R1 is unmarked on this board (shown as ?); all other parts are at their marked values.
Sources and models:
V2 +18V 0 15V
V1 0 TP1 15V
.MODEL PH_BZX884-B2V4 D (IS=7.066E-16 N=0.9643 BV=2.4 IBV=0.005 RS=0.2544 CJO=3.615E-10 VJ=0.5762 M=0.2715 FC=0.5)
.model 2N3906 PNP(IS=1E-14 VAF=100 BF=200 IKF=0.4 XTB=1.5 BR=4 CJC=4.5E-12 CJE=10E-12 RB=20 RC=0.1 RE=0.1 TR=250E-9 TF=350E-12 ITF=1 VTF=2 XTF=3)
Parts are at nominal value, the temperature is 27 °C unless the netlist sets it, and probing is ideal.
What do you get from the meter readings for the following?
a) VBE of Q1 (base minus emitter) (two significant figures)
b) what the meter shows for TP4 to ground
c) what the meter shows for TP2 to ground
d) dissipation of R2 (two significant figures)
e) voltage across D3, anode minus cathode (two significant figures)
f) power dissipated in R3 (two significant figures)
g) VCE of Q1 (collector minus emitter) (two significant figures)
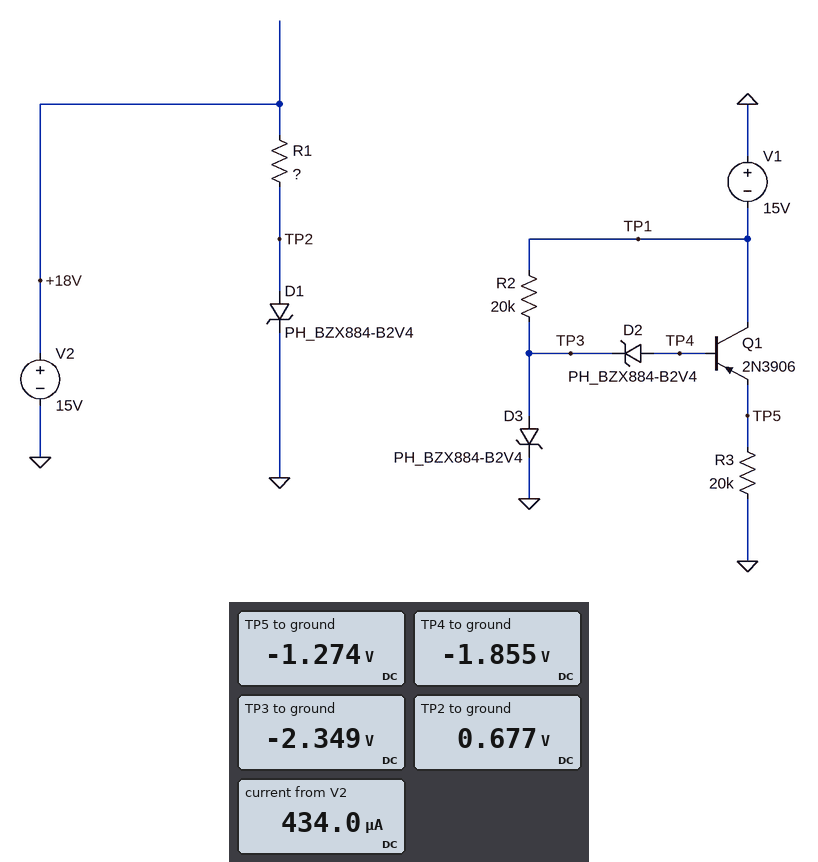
-580 mV
-1.855 V
0.677 V
8.0 mW
-2.3 V
81 µW
-14 V
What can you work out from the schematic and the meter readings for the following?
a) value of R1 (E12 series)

33 kΩ
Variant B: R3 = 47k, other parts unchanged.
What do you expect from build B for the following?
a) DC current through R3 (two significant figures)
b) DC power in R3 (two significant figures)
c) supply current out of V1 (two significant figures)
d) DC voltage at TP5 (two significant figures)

28 µA
37 µW
660 µA
-1.3 V
